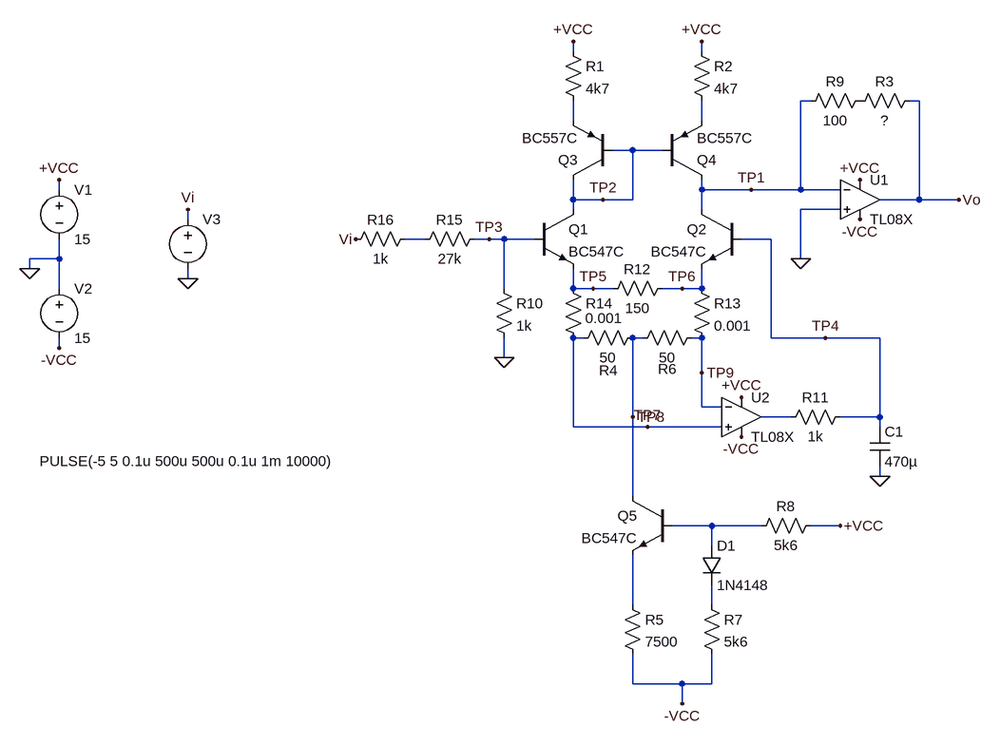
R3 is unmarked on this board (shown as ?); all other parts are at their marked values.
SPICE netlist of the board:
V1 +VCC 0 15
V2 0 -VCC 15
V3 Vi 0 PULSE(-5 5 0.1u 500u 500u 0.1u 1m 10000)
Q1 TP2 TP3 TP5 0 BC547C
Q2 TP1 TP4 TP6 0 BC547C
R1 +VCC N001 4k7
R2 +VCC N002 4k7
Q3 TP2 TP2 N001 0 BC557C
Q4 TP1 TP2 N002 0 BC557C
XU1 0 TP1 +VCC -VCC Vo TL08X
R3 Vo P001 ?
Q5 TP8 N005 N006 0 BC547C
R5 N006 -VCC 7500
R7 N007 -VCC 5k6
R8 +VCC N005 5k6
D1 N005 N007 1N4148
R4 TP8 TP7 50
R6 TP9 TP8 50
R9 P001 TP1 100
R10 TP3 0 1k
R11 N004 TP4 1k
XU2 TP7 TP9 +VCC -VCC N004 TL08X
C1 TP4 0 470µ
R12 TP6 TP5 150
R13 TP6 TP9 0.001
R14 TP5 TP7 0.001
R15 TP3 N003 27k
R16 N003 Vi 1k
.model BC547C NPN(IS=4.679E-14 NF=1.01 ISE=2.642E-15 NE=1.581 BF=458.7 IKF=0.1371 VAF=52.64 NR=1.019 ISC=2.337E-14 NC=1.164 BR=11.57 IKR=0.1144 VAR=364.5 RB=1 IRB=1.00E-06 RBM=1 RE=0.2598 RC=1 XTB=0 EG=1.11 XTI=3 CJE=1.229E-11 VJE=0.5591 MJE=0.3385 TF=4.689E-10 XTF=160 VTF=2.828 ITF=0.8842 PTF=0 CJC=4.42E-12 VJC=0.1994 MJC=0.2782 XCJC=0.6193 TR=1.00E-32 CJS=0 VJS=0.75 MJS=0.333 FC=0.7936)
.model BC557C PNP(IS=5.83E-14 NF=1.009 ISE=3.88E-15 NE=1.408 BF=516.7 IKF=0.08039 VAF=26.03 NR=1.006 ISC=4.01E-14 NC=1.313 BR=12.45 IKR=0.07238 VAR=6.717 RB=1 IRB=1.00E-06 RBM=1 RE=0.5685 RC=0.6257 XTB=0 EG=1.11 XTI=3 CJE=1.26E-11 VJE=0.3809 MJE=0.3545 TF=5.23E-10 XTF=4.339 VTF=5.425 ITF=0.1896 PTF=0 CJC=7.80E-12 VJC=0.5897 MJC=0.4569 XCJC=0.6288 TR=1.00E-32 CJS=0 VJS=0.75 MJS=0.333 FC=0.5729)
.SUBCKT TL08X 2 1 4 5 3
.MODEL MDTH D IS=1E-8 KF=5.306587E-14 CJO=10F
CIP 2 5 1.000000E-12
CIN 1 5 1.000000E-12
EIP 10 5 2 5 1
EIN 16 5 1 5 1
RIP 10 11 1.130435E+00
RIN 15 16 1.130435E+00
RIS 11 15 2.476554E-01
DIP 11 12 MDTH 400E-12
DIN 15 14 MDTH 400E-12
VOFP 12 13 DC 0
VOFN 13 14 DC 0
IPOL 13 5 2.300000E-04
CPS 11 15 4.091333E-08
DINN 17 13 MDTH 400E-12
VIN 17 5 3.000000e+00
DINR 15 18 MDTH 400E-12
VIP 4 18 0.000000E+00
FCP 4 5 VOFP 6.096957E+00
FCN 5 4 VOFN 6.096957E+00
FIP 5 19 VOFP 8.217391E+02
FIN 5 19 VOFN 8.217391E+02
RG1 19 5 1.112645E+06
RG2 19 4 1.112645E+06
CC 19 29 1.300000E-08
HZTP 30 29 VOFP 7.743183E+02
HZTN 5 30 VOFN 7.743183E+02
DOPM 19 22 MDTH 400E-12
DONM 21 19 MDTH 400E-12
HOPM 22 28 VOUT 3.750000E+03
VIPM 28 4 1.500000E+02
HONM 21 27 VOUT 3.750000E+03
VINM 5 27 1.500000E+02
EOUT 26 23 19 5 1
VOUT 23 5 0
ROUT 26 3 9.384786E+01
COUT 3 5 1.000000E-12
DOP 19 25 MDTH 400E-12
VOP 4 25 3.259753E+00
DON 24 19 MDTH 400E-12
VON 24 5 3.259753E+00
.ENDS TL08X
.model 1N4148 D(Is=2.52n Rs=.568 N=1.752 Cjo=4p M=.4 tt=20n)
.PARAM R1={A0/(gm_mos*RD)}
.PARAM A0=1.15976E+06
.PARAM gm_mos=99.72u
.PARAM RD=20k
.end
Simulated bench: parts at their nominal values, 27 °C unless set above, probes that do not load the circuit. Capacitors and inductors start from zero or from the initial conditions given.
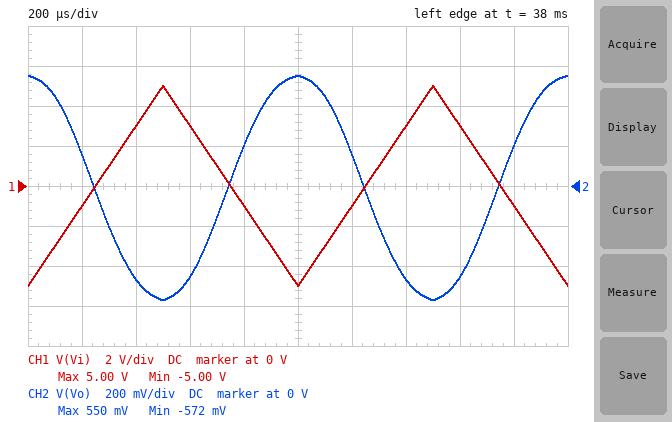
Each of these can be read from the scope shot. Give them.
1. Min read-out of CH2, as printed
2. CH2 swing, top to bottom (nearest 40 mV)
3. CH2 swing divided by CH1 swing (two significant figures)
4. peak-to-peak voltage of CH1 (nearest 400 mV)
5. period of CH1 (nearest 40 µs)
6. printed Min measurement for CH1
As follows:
-572 mV
1.12 V
0.11
10.0 V
1.00 ms
-5.00 V
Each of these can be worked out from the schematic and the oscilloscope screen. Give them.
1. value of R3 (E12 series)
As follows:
220 Ω
